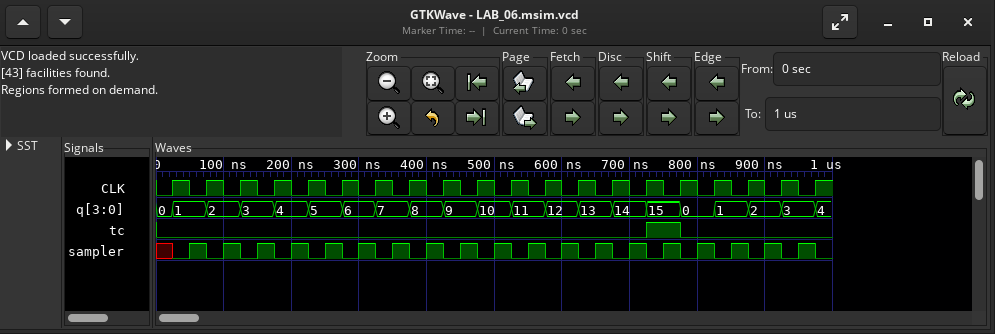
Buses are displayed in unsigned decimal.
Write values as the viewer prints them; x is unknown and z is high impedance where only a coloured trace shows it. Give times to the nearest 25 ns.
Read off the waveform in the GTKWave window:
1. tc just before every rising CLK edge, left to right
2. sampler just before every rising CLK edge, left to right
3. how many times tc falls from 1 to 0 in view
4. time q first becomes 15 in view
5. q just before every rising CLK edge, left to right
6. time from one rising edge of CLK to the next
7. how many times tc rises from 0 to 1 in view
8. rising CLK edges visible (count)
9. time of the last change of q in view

0 0 0 0 0 0 0 0 0 0 0 0 0 0 0 1 0 0 0 0
x 1 1 1 1 1 1 1 1 1 1 1 1 1 1 1 1 1 1 1
1
725 ns
0, 1, 2, 3, 4, 5, 6, 7, 8, 9, 10, 11, 12, 13, 14, 15, 0, 1, 2, 3
50 ns
1
20
975 ns
